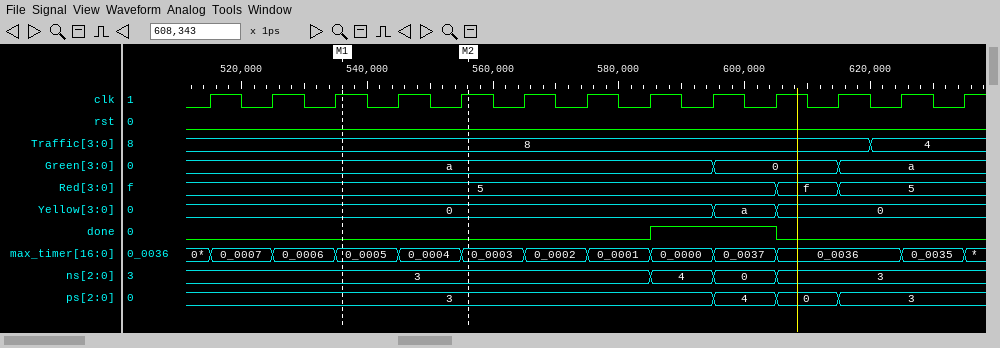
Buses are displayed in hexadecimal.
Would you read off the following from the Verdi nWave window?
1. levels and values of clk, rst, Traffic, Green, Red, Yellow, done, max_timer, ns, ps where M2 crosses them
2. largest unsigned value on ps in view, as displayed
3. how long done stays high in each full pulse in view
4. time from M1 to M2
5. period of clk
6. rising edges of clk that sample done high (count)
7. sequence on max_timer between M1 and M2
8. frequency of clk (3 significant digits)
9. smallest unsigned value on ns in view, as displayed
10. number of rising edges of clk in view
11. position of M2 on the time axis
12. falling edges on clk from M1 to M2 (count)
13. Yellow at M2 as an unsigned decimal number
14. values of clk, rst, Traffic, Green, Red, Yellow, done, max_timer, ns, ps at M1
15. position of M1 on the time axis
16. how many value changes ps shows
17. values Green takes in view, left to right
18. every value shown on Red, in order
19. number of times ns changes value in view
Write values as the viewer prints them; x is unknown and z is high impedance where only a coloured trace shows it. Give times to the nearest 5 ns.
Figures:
clk=1, rst=0, Traffic=8, Green=a, Red=5, Yellow=0, done=0, max_timer=0_0003, ns=3, ps=3
4
20 ns
20 ns
10 ns
2
0_0005, 0_0004, 0_0003
100 MHz
0
13
555 ns
2
0
clk=1, rst=0, Traffic=8, Green=a, Red=5, Yellow=0, done=0, max_timer=0_0005, ns=3, ps=3
535 ns
3
a, 0, a
5, f, 5
3
